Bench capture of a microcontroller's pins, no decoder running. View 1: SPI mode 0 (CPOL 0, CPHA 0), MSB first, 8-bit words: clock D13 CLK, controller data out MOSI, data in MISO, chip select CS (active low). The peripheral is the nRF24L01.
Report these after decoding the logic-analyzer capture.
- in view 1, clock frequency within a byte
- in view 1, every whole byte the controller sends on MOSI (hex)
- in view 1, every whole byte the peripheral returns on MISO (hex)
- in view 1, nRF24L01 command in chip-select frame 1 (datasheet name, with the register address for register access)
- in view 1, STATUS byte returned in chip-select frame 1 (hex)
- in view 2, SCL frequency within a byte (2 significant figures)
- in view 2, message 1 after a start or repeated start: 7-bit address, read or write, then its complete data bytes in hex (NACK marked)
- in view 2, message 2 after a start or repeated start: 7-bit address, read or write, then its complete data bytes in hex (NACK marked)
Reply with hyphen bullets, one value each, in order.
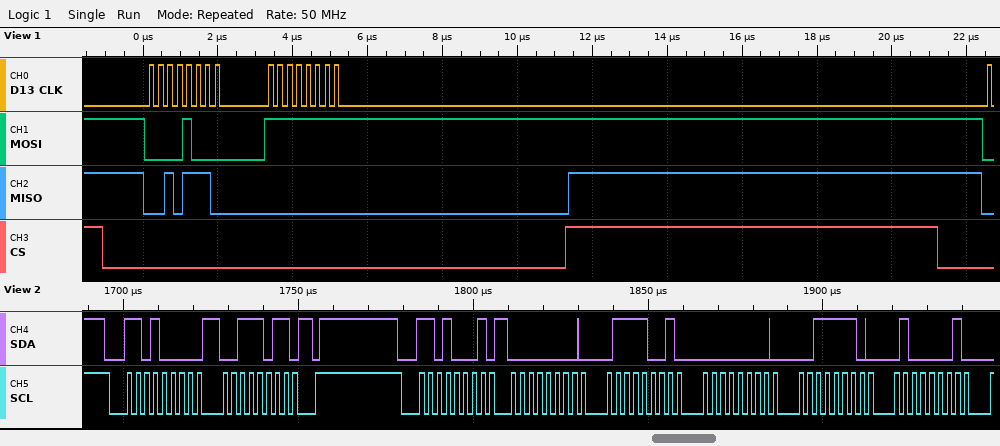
- 4 MHz
- 08 FF
- 2E 00
- R_REGISTER 0x08
- 0x2E
- 400 kHz
- 0x68 write: 3B
- 0x68 read: 00 79 00 3E 41
